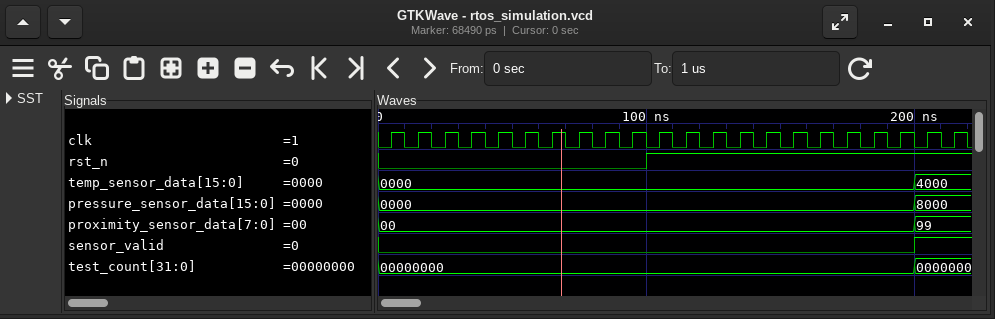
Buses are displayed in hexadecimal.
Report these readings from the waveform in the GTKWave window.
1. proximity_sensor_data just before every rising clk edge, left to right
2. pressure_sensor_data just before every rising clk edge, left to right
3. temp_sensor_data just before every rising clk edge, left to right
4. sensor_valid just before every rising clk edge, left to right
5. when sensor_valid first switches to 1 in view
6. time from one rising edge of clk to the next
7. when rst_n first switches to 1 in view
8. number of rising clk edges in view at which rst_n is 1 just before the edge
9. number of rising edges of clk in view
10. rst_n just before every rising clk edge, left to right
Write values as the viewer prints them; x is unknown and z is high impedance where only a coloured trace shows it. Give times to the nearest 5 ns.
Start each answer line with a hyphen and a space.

- 00, 00, 00, 00, 00, 00, 00, 00, 00, 00, 00, 00, 00, 00, 00, 00, 00, 00, 00, 00, 99, 99
- 0000, 0000, 0000, 0000, 0000, 0000, 0000, 0000, 0000, 0000, 0000, 0000, 0000, 0000, 0000, 0000, 0000, 0000, 0000, 0000, 8000, 8000
- 0000, 0000, 0000, 0000, 0000, 0000, 0000, 0000, 0000, 0000, 0000, 0000, 0000, 0000, 0000, 0000, 0000, 0000, 0000, 0000, 4000, 4000
- 0 0 0 0 0 0 0 0 0 0 0 0 0 0 0 0 0 0 0 0 1 1
- 200 ns
- 10 ns
- 100 ns
- 12
- 22
- 0 0 0 0 0 0 0 0 0 0 1 1 1 1 1 1 1 1 1 1 1 1
